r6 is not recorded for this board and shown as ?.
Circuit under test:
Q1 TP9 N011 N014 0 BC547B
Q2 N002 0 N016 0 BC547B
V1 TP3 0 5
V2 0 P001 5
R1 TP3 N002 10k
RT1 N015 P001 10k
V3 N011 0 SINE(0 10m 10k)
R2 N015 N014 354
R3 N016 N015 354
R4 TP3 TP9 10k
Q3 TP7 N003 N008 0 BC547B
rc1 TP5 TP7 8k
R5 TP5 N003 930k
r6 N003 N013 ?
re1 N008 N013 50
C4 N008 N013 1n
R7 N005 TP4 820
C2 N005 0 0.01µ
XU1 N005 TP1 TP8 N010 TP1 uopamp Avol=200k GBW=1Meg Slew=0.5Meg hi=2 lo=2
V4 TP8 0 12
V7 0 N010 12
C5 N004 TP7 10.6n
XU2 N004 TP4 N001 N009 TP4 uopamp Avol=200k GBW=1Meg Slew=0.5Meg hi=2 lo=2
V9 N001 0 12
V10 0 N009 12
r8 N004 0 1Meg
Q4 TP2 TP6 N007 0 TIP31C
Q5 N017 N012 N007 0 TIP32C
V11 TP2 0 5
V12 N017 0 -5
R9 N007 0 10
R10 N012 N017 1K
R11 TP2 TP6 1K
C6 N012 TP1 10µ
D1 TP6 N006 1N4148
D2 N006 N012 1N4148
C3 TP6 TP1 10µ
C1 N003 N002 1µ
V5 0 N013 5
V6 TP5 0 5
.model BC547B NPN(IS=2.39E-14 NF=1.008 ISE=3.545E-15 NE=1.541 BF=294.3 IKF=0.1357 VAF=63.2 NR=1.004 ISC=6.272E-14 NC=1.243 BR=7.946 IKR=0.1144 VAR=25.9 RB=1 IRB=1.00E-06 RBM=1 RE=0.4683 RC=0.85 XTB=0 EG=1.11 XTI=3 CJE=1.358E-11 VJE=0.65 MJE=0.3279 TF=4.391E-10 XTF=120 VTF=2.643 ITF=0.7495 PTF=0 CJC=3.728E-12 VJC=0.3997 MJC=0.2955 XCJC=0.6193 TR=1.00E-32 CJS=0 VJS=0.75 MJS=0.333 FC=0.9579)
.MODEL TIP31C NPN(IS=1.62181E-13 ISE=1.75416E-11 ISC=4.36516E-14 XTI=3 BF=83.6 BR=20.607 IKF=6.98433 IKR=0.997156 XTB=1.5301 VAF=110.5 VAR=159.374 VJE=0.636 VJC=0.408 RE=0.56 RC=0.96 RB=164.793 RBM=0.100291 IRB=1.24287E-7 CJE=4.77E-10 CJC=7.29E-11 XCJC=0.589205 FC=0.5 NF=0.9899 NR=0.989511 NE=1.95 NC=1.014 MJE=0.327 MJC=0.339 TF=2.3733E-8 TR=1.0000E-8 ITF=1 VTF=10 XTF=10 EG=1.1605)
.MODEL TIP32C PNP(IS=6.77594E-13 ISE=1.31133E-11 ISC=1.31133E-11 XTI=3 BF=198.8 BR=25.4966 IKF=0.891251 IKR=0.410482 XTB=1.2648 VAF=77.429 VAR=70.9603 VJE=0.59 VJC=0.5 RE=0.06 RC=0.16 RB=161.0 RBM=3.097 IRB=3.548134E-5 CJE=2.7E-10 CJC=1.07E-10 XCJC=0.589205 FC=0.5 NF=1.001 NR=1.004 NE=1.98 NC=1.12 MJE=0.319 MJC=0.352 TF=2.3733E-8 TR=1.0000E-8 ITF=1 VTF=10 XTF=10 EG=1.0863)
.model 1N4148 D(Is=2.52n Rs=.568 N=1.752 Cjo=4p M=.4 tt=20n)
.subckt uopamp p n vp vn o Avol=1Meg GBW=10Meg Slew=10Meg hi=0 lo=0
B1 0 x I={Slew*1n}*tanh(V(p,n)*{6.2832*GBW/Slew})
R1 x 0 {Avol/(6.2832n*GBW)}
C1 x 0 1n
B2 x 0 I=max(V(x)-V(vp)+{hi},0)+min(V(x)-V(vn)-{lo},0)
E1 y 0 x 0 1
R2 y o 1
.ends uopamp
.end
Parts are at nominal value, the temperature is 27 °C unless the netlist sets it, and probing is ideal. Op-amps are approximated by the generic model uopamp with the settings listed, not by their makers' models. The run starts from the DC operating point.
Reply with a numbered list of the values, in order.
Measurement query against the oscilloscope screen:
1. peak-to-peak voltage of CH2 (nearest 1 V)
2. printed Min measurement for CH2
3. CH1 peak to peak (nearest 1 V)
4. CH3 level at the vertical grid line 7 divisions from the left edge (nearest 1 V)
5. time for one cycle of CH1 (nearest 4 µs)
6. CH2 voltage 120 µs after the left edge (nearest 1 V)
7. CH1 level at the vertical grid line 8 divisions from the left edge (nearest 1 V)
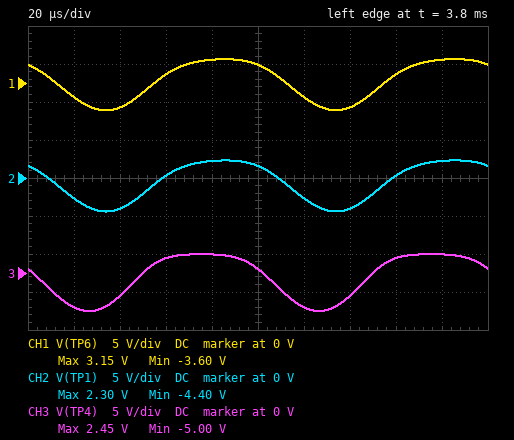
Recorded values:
1. 7 V
2. -4.40 V
3. 7 V
4. -3 V
5. 100 µs
6. -3 V
7. 1 V
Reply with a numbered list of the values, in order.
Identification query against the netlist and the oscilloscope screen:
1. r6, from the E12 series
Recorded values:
1. 68 kΩ
